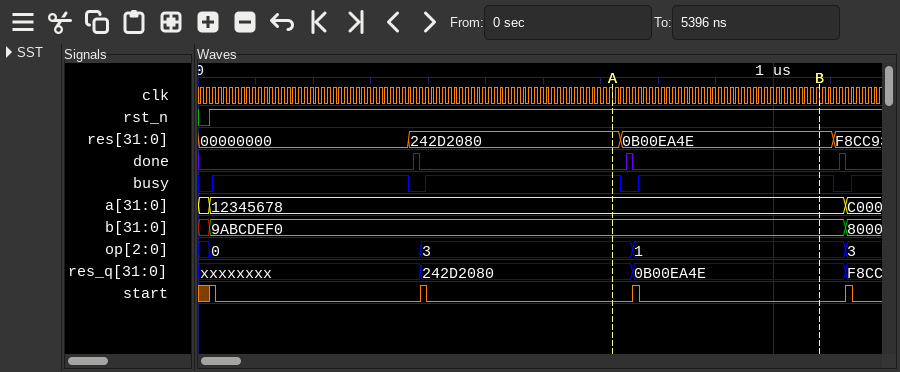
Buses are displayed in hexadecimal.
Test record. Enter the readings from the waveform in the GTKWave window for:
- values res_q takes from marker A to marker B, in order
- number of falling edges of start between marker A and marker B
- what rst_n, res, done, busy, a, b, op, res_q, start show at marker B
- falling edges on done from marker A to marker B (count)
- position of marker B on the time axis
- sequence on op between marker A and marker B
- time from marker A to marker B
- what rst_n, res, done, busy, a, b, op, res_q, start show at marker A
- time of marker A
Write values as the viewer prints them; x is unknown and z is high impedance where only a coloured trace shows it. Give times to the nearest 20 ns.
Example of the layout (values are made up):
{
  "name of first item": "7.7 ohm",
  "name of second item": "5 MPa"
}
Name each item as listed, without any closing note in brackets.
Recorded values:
{
  "values res_q takes from marker A to marker B, in order": "242D2080, 0B00EA4E",
  "number of falling edges of start between marker A and marker B": "1",
  "what rst_n, res, done, busy, a, b, op, res_q, start show at marker B": "rst_n=1, res=0B00EA4E, done=0, busy=1, a=12345678, b=9ABCDEF0, op=1, res_q=0B00EA4E, start=0",
  "falling edges on done from marker A to marker B": "1",
  "position of marker B on the time axis": "1080 ns",
  "sequence on op between marker A and marker B": "3, 1",
  "time from marker A to marker B": "360 ns",
  "what rst_n, res, done, busy, a, b, op, res_q, start show at marker A": "rst_n=1, res=242D2080, done=0, busy=1, a=12345678, b=9ABCDEF0, op=3, res_q=242D2080, start=0",
  "time of marker A": "720 ns"
}
